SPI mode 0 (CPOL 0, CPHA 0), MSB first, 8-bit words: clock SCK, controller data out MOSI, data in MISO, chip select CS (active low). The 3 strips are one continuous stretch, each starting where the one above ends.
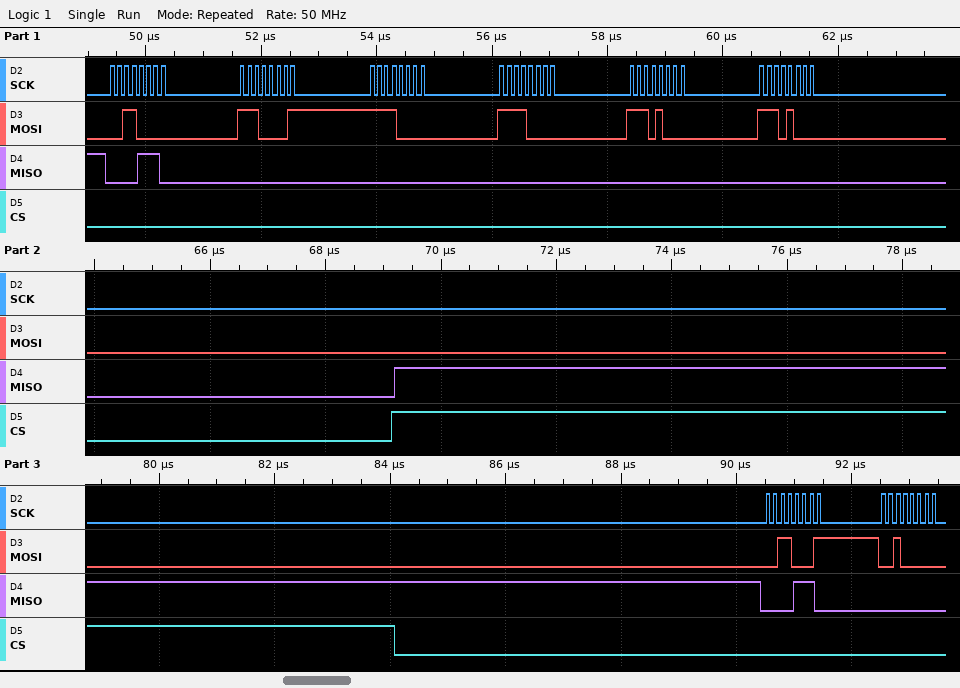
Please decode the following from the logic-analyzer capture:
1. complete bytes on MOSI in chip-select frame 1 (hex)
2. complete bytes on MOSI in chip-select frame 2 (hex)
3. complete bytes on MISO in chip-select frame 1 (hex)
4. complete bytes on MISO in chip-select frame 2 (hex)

30 E1 F0 F0 E8 E8
31 20
0E 00 00 00 00 00
0E 00
